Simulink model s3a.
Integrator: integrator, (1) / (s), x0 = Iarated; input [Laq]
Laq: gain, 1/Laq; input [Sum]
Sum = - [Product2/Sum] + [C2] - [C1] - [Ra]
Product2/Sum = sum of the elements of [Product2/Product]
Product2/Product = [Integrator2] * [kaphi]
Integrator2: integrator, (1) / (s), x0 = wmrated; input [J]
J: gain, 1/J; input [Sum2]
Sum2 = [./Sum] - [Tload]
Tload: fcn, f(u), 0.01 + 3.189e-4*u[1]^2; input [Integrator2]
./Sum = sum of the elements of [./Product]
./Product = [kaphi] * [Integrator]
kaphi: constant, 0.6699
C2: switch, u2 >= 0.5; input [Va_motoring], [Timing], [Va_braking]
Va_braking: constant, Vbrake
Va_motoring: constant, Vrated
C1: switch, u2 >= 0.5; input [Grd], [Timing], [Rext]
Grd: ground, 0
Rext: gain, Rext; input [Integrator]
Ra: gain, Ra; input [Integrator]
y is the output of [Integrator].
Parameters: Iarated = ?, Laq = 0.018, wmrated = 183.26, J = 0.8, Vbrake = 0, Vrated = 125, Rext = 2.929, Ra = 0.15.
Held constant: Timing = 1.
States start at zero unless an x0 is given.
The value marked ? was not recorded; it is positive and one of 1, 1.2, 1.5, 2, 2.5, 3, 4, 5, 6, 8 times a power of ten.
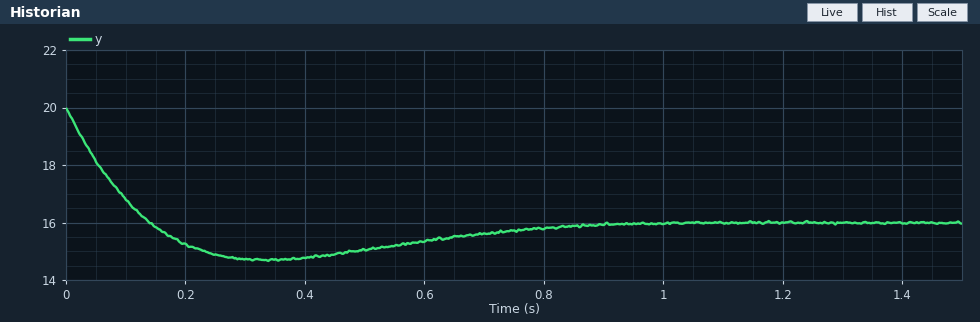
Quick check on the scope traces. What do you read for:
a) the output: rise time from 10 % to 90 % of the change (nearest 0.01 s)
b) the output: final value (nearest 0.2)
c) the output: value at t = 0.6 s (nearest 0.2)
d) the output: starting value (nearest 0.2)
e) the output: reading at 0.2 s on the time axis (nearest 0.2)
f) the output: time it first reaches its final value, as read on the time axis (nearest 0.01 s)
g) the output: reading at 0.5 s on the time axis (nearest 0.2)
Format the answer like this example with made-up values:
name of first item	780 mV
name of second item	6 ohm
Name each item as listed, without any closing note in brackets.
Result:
the output: rise time from 10 % to 90 % of the change	0.11 s
the output: final value	16.0
the output: value at t = 0.6 s	15.4
the output: starting value	20.0
the output: reading at 0.2 s on the time axis	15.2
the output: time it first reaches its final value, as read on the time axis	0.14 s
the output: reading at 0.5 s on the time axis	15.0
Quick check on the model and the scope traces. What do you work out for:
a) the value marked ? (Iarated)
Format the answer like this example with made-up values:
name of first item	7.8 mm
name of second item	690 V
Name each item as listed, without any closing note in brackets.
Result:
the value marked ?	20
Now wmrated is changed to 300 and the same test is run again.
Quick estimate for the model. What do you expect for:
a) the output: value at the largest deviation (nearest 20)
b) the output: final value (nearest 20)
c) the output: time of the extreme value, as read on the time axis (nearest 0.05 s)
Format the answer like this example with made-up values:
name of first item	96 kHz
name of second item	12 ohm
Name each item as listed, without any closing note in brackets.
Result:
the output: value at the largest deviation	-320
the output: final value	20
the output: time of the extreme value, as read on the time axis	0.20 s
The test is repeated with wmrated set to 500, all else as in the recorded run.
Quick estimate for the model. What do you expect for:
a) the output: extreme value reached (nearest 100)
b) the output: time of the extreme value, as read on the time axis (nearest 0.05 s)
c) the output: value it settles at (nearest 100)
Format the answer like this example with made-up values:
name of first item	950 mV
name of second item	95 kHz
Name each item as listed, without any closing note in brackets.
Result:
the output: extreme value reached	-900
the output: time of the extreme value, as read on the time axis	0.20 s
the output: value it settles at	0
